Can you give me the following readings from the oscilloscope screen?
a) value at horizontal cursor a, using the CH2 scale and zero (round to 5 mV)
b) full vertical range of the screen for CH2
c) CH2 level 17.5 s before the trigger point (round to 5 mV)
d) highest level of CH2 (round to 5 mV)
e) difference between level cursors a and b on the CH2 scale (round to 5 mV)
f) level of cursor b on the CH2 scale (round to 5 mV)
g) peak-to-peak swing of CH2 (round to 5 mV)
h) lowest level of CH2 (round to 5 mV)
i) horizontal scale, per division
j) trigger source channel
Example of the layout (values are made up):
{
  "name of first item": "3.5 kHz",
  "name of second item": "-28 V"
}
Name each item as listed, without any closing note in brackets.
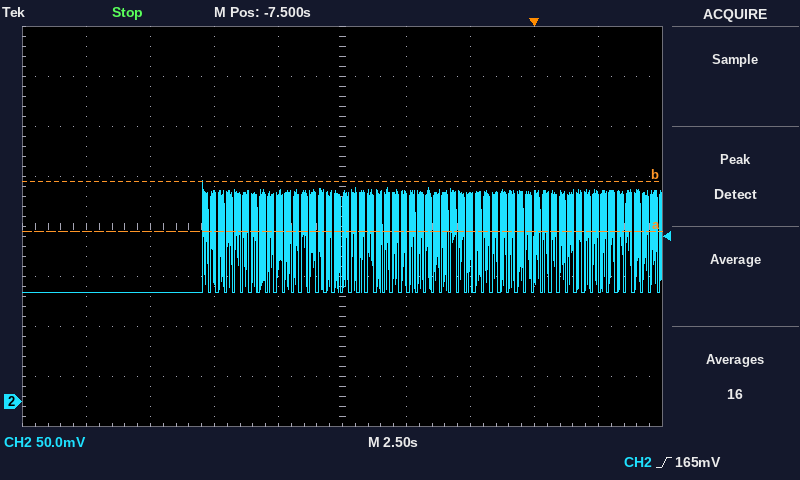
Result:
{
  "value at horizontal cursor a, using the CH2 scale and zero": "170 mV",
  "full vertical range of the screen for CH2": "400 mV",
  "CH2 level 17.5 s before the trigger point": "110 mV",
  "highest level of CH2": "220 mV",
  "difference between level cursors a and b on the CH2 scale": "50 mV",
  "level of cursor b on the CH2 scale": "220 mV",
  "peak-to-peak swing of CH2": "110 mV",
  "lowest level of CH2": "110 mV",
  "horizontal scale, per division": "2.5 s",
  "trigger source channel": "CH2"
}
